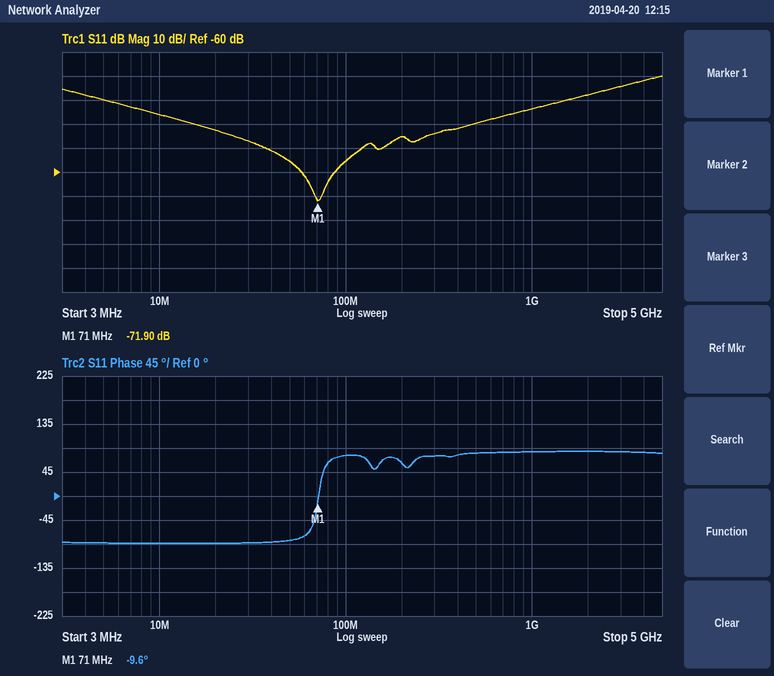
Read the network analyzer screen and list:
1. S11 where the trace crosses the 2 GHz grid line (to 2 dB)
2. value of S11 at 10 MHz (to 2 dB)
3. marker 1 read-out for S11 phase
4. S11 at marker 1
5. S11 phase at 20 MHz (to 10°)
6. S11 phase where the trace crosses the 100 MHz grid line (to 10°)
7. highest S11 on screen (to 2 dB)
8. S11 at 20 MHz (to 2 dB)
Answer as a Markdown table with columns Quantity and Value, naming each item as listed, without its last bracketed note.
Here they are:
| Quantity | Value |
|---|---|
| S11 where the trace crosses the 2 GHz grid line | -28 dB |
| value of S11 at 10 MHz | -36 dB |
| marker 1 read-out for S11 phase | -9.6° |
| S11 at marker 1 | -71.90 dB |
| S11 phase at 20 MHz | -90° |
| S11 phase where the trace crosses the 100 MHz grid line | 80° |
| highest S11 on screen | -20 dB |
| S11 at 20 MHz | -42 dB |
